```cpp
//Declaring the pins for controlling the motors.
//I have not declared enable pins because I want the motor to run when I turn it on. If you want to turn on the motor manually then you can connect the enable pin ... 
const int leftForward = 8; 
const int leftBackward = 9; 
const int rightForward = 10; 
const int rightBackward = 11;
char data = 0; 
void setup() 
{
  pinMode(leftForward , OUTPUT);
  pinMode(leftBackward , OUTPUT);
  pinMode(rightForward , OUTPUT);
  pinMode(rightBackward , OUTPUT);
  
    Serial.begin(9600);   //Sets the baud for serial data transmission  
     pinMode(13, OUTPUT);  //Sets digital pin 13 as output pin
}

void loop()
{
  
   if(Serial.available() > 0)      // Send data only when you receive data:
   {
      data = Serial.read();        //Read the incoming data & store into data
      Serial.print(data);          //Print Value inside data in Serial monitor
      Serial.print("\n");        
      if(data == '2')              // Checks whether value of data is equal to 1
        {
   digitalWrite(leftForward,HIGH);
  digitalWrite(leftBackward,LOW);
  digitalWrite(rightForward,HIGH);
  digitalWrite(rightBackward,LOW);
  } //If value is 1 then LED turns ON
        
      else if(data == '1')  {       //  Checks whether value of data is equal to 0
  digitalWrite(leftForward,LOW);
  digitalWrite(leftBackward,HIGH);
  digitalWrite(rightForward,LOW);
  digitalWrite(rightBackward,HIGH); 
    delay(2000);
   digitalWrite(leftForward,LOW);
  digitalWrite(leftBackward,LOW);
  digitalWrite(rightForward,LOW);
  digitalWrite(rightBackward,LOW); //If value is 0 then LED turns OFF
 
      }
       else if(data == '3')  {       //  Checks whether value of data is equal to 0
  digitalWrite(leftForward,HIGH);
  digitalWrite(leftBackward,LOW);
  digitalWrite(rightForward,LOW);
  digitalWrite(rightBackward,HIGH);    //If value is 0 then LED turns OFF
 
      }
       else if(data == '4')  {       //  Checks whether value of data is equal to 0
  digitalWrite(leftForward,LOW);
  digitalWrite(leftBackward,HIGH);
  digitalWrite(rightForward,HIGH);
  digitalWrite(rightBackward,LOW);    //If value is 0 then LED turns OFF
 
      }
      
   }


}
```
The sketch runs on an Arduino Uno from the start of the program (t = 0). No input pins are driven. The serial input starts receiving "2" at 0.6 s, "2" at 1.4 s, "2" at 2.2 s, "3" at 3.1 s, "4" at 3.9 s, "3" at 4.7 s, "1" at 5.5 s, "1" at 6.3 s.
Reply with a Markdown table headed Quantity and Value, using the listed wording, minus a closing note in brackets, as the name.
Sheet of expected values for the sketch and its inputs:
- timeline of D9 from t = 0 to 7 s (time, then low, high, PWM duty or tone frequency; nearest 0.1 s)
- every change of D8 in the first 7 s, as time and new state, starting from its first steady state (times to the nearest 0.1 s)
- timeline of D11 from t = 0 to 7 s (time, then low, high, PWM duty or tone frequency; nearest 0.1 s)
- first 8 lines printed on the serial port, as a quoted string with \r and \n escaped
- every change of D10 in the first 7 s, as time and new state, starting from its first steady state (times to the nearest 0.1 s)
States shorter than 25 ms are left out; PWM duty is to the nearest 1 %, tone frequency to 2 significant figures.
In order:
| Quantity | Value |
|---|---|
| timeline of D9 from t = 0 to 7 s | 0 s low; 3.9 s high; 4.7 s low; 5.5 s high |
| every change of D8 in the first 7 s, as time and new state, starting from its first steady state | 0 s low; 0.6 s high; 3.9 s low; 4.7 s high; 5.5 s low |
| timeline of D11 from t = 0 to 7 s | 0 s low; 3.1 s high; 3.9 s low; 4.7 s high |
| first 8 lines printed on the serial port, as a quoted string with \r and \n escaped | "2\n2\n2\n3\n4\n3\n1\n1\n" |
| every change of D10 in the first 7 s, as time and new state, starting from its first steady state | 0 s low; 0.6 s high; 3.1 s low; 3.9 s high; 4.7 s low |
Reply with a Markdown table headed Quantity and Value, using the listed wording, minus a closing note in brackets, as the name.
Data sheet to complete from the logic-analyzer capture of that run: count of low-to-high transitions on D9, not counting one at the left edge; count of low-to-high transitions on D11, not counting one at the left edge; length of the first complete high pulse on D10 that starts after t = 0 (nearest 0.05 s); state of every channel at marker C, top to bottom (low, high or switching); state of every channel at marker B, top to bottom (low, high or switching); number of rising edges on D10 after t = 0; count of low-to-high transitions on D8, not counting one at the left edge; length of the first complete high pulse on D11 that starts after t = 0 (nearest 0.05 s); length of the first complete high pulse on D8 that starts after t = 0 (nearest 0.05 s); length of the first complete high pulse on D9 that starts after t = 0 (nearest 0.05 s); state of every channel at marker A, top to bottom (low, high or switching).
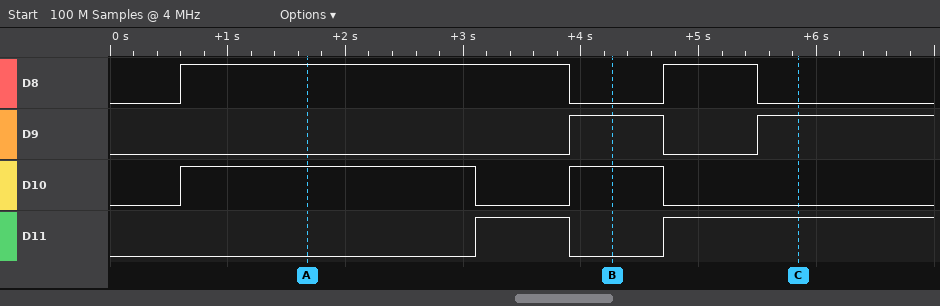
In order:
| Quantity | Value |
|---|---|
| count of low-to-high transitions on D9, not counting one at the left edge | 2 |
| count of low-to-high transitions on D11, not counting one at the left edge | 2 |
| length of the first complete high pulse on D10 that starts after t = 0 | 2.50 s |
| state of every channel at marker C, top to bottom | D8 low, D9 high, D10 low, D11 high |
| state of every channel at marker B, top to bottom | D8 low, D9 high, D10 high, D11 low |
| number of rising edges on D10 after t = 0 | 2 |
| count of low-to-high transitions on D8, not counting one at the left edge | 2 |
| length of the first complete high pulse on D11 that starts after t = 0 | 0.80 s |
| length of the first complete high pulse on D8 that starts after t = 0 | 3.30 s |
| length of the first complete high pulse on D9 that starts after t = 0 | 0.80 s |
| state of every channel at marker A, top to bottom | D8 high, D9 low, D10 high, D11 low |
